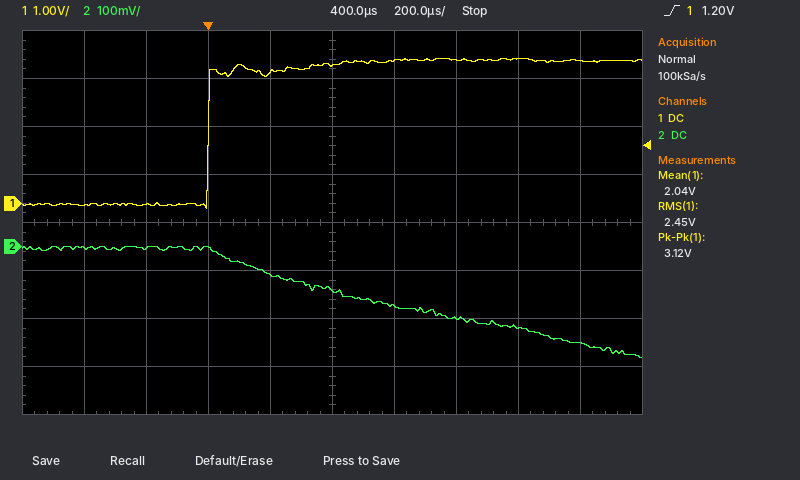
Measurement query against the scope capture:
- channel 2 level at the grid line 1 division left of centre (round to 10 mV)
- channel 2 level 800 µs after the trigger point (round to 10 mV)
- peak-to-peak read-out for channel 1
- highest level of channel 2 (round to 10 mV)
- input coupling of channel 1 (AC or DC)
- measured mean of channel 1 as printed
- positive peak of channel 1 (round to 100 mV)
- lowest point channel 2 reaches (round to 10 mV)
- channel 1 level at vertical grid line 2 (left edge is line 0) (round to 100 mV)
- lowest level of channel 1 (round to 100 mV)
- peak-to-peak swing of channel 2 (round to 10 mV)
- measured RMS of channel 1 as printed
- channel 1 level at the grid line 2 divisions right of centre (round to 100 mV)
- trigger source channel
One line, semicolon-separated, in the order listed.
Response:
-60 mV; -150 mV; 3.12 V; 0 mV; DC; 2.04 V; 3.0 V; -230 mV; 0.0 V; -100 mV; 230 mV; 2.45 V; 3.0 V; channel 1
